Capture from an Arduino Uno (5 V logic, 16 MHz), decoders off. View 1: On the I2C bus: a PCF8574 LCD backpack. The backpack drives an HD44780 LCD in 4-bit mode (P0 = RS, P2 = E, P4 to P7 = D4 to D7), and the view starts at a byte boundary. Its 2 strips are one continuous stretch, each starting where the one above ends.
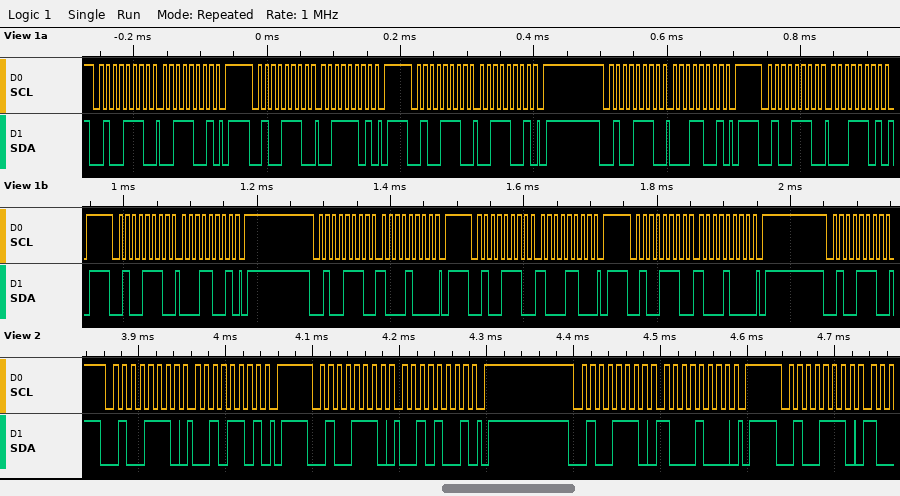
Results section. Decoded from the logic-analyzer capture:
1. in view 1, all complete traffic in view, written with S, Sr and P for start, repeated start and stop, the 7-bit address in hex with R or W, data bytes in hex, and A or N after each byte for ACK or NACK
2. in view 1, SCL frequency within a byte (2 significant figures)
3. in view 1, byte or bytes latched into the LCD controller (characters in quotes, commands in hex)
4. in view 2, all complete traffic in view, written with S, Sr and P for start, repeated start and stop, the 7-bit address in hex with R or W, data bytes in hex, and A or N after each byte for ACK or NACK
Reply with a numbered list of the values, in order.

1. S 27W A 39 A P S 27W A 3D A P S 27W A 39 A P S 27W A 19 A P S 27W A 1D A P S 27W A 19 A P S 27W A 88 A P S 27W A 8C A P S 27W A 88 A P S 27W A
2. 100 kHz
3. '1'
4. S 27W A 2D A P S 27W A 29 A P S 27W A 88 A P S 27W A
